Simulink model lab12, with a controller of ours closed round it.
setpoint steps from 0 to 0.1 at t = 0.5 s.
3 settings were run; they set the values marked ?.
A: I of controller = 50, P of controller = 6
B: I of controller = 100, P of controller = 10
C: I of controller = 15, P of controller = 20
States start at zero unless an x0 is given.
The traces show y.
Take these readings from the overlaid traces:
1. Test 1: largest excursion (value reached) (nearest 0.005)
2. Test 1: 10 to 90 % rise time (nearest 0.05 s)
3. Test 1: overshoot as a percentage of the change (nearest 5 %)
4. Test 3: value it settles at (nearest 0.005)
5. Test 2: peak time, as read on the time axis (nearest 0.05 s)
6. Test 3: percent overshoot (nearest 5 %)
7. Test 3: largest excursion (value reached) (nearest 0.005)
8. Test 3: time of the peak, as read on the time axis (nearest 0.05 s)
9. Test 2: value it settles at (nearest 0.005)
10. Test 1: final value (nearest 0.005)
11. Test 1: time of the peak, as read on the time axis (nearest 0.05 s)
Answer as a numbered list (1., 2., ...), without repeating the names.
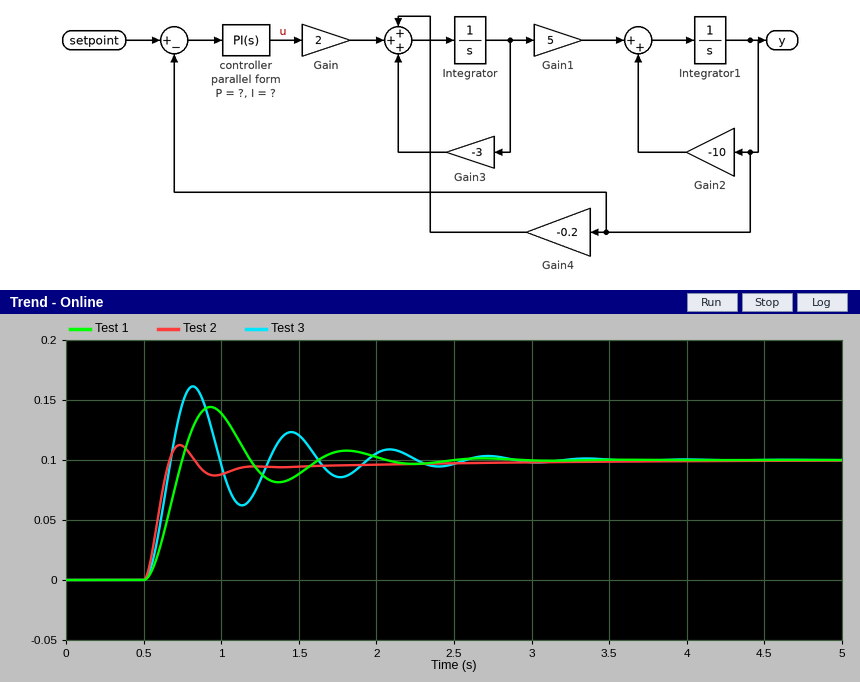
1. 0.145
2. 0.15 s
3. 45 %
4. 0.100
5. 0.75 s
6. 60 %
7. 0.160
8. 0.80 s
9. 0.100
10. 0.100
11. 0.95 s
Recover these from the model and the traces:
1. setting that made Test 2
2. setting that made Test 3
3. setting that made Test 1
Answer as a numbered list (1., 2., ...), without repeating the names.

1. C
2. B
3. A
